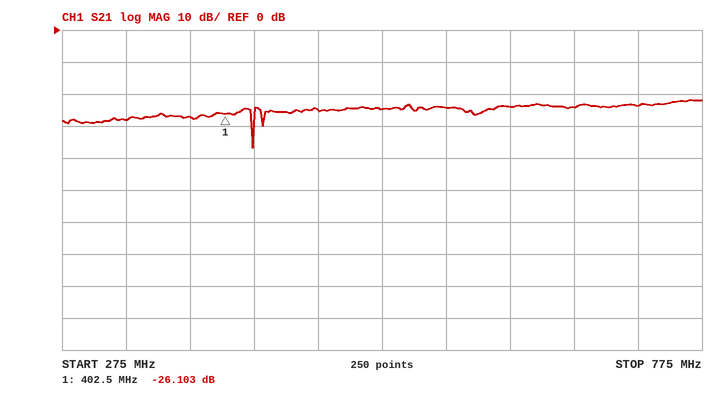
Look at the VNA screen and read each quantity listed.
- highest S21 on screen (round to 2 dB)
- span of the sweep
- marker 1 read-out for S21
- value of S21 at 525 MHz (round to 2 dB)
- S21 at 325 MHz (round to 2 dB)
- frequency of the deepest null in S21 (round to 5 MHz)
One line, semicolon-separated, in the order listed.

-22 dB; 500 MHz; -26.103 dB; -24 dB; -28 dB; 425 MHz
